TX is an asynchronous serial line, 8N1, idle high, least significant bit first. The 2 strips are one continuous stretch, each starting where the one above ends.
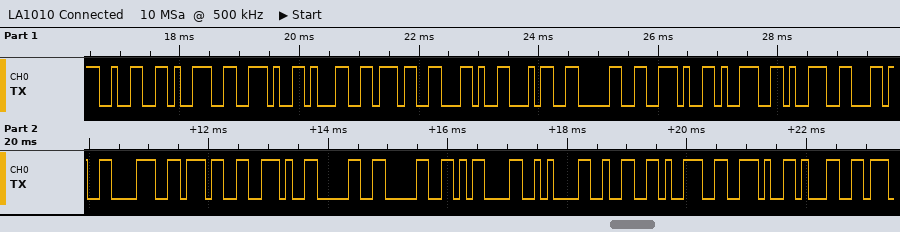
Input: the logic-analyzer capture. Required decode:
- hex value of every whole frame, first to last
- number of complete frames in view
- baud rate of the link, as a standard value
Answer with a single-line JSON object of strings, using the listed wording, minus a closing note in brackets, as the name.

{"hex value of every whole frame, first to last": "32 39 2E 31 37 2C 34 30 2E 39 39 2C 38 37 2E 30 30 0D 0A 32 39 2E 31", "number of complete frames in view": "23", "baud rate of the link, as a standard value": "9600 baud"}
